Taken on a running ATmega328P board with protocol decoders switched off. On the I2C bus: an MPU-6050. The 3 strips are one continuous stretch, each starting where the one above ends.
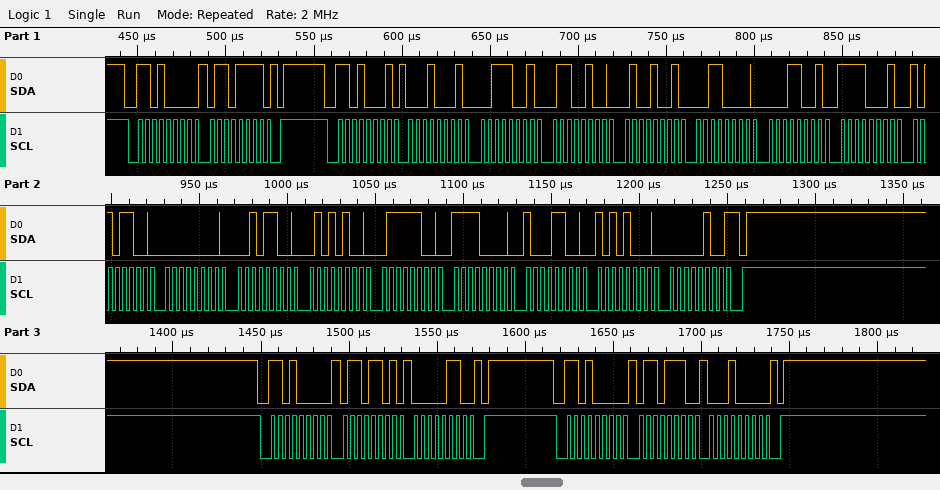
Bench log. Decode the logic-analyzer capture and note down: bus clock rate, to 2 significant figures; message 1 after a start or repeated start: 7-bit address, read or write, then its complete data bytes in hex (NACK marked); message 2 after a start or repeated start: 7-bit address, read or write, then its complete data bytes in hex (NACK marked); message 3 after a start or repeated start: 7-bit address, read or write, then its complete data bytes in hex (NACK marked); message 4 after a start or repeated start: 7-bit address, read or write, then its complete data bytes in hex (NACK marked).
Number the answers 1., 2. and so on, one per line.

1. 250 kHz
2. 0x68 write: 6F
3. 0x68 read: 11 39 64 49 30 19 F1 AC 00 2C 54 7C F0 8C A8 04 NACK
4. 0x68 write: 6D 06
5. 0x68 write: 6E 10
